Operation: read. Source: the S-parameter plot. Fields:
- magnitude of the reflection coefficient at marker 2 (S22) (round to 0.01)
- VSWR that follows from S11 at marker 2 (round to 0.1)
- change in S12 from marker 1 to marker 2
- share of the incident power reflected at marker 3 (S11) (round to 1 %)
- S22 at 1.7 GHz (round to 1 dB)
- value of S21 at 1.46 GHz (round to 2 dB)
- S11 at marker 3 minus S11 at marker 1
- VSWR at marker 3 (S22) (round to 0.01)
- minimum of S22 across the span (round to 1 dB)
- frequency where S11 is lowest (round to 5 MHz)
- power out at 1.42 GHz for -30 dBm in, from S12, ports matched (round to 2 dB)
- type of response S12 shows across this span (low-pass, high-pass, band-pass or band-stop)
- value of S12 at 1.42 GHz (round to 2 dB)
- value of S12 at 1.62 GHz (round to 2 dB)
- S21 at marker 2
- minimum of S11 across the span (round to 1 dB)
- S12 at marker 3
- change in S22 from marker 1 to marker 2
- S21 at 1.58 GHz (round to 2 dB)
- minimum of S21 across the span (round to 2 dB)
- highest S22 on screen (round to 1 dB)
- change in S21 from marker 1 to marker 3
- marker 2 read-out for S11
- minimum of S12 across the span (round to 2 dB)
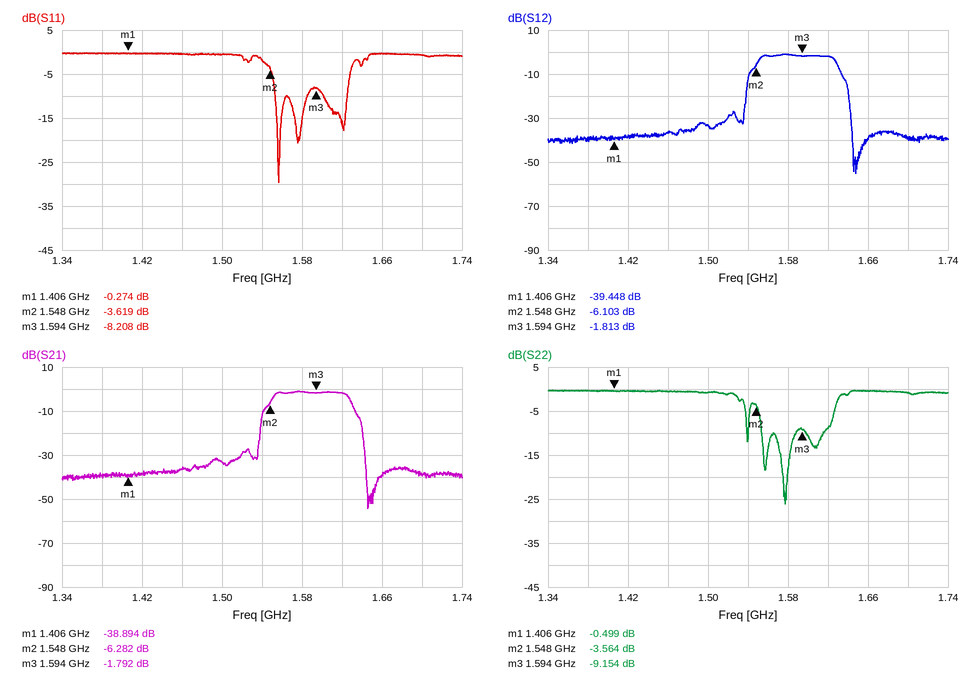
0.66
4.9
33.345 dB
15 %
-1 dB
-36 dB
-7.934 dB
2.07
-26 dB
1.555 GHz
-68 dBm
band-pass
-38 dB
-2 dB
-6.282 dB
-30 dB
-1.813 dB
-3.065 dB
-2 dB
-54 dB
0 dB
37.102 dB
-3.619 dB
-56 dB
